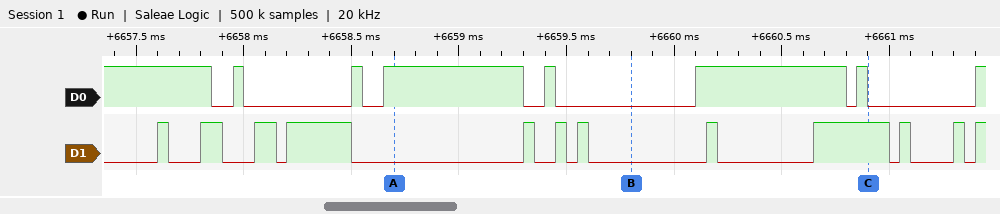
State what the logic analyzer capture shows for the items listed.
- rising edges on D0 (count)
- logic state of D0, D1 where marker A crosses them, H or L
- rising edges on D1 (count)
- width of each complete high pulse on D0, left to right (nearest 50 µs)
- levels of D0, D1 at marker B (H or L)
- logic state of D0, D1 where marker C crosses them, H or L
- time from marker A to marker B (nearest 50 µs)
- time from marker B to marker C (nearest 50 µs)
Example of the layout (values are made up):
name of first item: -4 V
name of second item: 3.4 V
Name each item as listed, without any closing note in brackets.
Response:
rising edges on D0: 7
logic state of D0, D1 where marker A crosses them, H or L: D0=H, D1=L
rising edges on D1: 12
width of each complete high pulse on D0, left to right: 50 µs, 50 µs, 650 µs, 50 µs, 700 µs, 50 µs
levels of D0, D1 at marker B: D0=L, D1=L
logic state of D0, D1 where marker C crosses them, H or L: D0=L, D1=H
time from marker A to marker B: 1100 µs
time from marker B to marker C: 1100 µs
